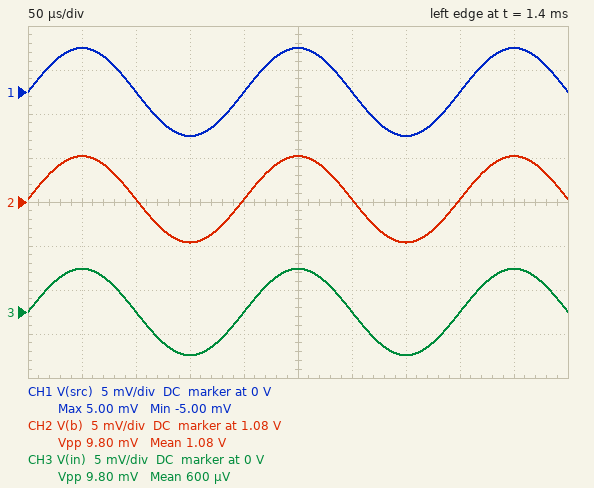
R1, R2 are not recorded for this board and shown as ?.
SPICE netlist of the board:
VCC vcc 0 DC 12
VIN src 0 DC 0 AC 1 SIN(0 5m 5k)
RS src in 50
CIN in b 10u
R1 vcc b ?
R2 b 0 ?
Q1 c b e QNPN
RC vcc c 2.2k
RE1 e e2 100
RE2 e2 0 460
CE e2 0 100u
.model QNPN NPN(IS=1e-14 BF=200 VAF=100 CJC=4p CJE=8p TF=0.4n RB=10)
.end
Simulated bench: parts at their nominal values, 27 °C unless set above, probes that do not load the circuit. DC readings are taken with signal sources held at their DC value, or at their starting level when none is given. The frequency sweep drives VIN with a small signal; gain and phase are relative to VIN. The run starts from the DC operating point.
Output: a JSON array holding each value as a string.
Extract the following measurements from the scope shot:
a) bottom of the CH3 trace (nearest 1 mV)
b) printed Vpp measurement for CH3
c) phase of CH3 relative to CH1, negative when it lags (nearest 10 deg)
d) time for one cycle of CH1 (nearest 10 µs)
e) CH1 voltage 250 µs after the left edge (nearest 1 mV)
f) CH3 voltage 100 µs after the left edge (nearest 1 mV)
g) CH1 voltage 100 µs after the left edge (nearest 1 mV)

["-5 mV", "9.80 mV", "0 deg", "200 µs", "5 mV", "0 V", "0 V"]
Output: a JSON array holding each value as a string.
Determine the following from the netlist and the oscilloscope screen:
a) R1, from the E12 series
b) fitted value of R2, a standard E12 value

["33 kΩ", "3.3 kΩ"]
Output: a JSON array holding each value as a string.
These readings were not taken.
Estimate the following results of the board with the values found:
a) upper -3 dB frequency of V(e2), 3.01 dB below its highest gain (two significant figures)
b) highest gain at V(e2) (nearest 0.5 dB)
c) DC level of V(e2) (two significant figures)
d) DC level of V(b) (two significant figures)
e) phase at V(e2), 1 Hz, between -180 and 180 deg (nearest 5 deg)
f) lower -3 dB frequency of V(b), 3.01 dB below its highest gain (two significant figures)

["24 Hz", "-5.0 dB", "360 mV", "1.1 V", "75 deg", "5.5 Hz"]
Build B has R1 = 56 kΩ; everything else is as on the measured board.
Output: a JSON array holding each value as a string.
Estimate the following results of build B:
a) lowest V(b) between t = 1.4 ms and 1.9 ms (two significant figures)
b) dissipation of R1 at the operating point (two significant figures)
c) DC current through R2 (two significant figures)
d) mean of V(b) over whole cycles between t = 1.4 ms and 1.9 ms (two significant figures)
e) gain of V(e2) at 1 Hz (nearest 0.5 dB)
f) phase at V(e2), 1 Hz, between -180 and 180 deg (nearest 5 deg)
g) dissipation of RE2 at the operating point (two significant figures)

["660 mV", "2.3 mW", "200 µA", "670 mV", "-19.0 dB", "70 deg", "6.8 µW"]
